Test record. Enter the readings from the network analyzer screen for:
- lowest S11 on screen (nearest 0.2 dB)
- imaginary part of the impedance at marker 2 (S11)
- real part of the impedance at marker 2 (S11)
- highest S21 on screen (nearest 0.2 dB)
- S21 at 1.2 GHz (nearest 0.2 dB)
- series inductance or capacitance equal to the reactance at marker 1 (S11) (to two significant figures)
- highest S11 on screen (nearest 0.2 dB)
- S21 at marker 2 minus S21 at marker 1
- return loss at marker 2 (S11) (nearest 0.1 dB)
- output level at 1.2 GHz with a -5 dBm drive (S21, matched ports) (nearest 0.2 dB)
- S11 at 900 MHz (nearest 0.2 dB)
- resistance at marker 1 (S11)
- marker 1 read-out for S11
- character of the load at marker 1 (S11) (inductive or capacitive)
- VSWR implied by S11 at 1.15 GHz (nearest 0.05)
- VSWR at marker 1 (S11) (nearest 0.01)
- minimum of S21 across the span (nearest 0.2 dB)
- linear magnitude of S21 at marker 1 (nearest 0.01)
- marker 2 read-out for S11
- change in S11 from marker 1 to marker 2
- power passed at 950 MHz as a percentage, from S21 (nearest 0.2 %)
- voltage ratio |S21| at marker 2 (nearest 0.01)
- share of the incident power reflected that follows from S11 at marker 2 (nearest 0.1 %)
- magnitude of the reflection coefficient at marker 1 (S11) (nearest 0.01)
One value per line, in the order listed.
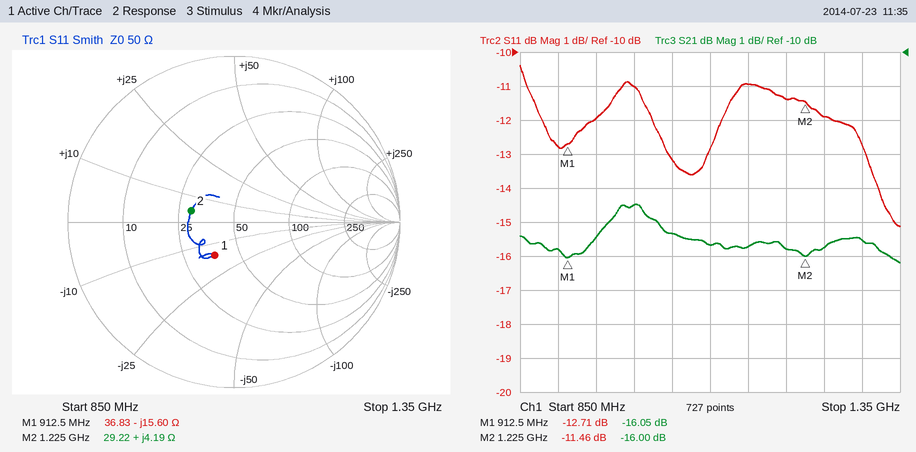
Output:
-15.2 dB
+4.19 Ω
29.22 Ω
-14.4 dB
-15.8 dB
11 pF
-10.4 dB
0.05 dB
11.5 dB
-20.8 dBm
-12.8 dB
36.83 Ω
-12.71 dB
capacitive
1.80
1.60
-16.2 dB
0.16
-11.46 dB
1.25 dB
2.8 %
0.16
7.1 %
0.23
